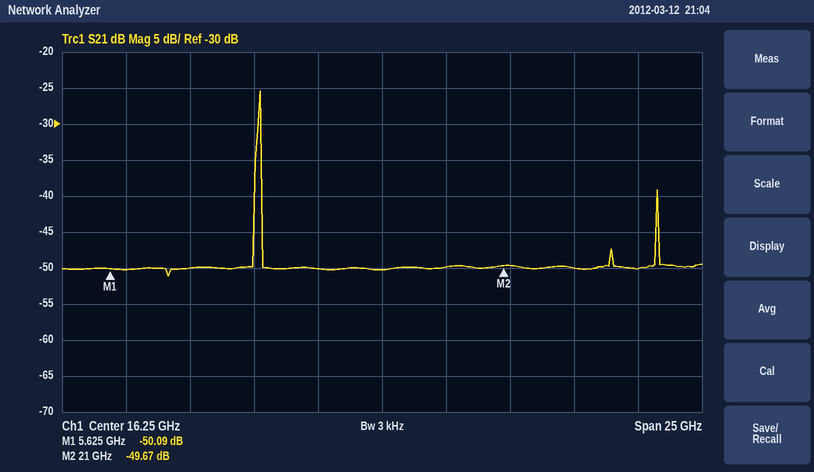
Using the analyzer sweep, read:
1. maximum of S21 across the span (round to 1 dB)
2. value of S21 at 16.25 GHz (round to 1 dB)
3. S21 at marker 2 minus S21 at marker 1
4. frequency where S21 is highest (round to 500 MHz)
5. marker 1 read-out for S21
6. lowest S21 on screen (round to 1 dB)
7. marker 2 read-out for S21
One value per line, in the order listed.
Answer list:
-25 dB
-50 dB
0.42 dB
11.5 GHz
-50.09 dB
-51 dB
-49.67 dB
